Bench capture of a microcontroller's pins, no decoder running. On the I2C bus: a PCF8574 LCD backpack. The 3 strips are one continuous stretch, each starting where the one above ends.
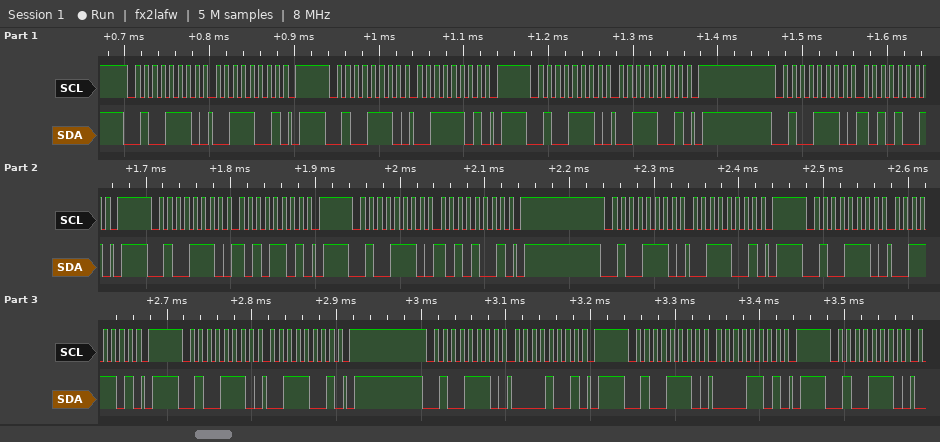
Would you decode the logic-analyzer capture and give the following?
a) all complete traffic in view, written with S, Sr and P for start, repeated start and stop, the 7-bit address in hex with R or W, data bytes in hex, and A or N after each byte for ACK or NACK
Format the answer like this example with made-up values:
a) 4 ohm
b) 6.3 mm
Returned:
a) S 27W A 39 A P S 27W A 3D A P S 27W A 39 A P S 27W A A9 A P S 27W A AD A P S 27W A A9 A P S 27W A 39 A P S 27W A 3D A P S 27W A 39 A P S 27W A 09 A P S 27W A 0D A P S 27W A
